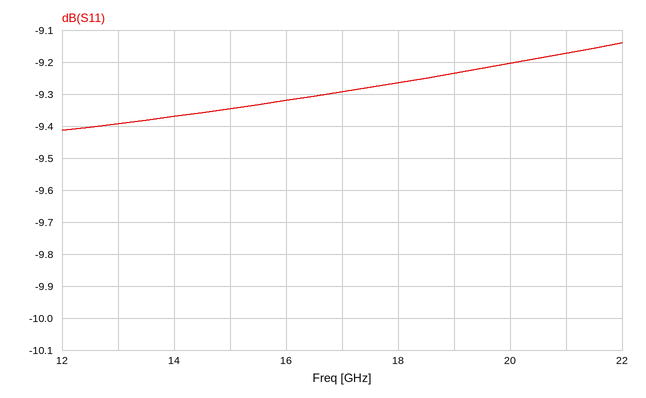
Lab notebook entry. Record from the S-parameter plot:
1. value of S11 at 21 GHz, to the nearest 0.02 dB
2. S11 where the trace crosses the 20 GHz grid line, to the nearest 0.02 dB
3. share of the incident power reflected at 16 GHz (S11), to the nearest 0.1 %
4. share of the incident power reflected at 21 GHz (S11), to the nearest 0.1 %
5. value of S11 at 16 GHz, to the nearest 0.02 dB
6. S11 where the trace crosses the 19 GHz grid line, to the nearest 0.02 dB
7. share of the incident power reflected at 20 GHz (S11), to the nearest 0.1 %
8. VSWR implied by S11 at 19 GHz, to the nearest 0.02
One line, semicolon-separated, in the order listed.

-9.18 dB; -9.20 dB; 11.7 %; 12.1 %; -9.32 dB; -9.24 dB; 12.0 %; 2.06
